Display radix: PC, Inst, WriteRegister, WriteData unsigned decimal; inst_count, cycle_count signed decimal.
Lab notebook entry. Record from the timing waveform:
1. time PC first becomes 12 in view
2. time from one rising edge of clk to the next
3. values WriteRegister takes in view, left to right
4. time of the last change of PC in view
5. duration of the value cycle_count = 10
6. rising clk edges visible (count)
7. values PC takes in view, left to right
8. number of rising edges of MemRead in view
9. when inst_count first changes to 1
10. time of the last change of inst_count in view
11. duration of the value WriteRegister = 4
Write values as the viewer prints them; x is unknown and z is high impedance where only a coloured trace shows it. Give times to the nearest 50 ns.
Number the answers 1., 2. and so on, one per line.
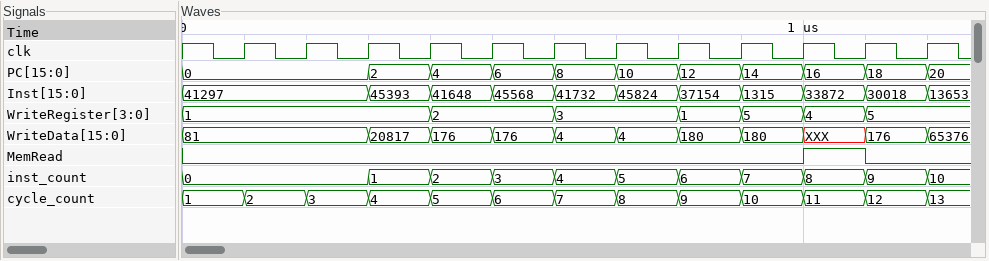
1. 800 ns
2. 100 ns
3. 1, 2, 3, 1, 5, 4, 5
4. 1200 ns
5. 100 ns
6. 12
7. 0, 2, 4, 6, 8, 10, 12, 14, 16, 18, 20
8. 1
9. 300 ns
10. 1200 ns
11. 100 ns
